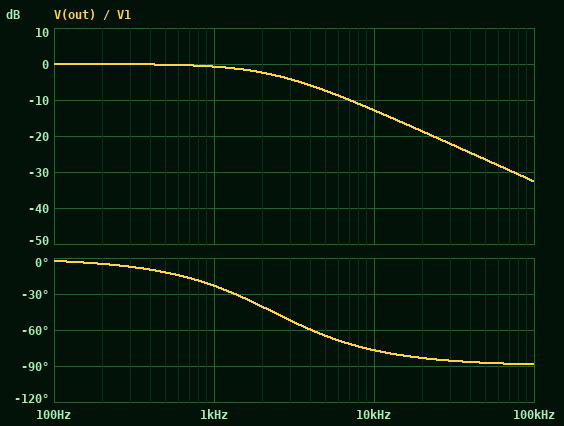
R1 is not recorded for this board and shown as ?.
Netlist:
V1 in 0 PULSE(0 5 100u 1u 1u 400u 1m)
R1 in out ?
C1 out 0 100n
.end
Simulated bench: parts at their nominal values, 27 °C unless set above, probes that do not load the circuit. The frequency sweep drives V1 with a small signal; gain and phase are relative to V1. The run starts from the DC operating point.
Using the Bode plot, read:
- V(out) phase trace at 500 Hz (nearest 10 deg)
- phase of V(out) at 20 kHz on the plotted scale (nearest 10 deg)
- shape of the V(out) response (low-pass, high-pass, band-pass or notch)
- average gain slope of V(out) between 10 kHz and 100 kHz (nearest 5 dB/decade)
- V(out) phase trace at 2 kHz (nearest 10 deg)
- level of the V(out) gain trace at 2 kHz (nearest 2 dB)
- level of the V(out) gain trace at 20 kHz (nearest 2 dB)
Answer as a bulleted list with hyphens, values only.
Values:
- -10 deg
- -80 deg
- low-pass
- -20 dB/decade
- -40 deg
- -2 dB
- -18 dB
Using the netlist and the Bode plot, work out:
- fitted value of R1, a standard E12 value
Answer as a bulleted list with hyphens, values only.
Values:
- 680 Ω
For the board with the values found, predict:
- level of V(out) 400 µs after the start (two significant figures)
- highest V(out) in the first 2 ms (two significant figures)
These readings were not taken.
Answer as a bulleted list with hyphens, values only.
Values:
- 4.9 V
- 5.0 V
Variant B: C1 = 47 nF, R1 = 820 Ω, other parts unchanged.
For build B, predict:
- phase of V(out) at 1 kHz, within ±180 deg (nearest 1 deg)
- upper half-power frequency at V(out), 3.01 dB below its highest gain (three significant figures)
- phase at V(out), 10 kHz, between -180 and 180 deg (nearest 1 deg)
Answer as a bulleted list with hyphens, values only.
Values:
- -14 deg
- 4.13 kHz
- -68 deg
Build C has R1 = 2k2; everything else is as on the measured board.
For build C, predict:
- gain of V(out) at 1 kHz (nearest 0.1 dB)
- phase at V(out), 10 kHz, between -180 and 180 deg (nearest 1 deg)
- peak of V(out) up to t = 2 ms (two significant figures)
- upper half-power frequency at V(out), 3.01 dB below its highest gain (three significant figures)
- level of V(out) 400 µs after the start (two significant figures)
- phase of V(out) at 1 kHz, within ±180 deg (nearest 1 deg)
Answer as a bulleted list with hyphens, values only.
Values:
- -4.6 dB
- -86 deg
- 4.2 V
- 723 Hz
- 3.7 V
- -54 deg
